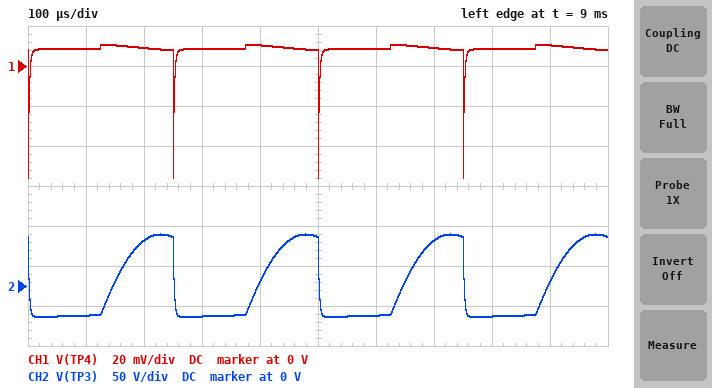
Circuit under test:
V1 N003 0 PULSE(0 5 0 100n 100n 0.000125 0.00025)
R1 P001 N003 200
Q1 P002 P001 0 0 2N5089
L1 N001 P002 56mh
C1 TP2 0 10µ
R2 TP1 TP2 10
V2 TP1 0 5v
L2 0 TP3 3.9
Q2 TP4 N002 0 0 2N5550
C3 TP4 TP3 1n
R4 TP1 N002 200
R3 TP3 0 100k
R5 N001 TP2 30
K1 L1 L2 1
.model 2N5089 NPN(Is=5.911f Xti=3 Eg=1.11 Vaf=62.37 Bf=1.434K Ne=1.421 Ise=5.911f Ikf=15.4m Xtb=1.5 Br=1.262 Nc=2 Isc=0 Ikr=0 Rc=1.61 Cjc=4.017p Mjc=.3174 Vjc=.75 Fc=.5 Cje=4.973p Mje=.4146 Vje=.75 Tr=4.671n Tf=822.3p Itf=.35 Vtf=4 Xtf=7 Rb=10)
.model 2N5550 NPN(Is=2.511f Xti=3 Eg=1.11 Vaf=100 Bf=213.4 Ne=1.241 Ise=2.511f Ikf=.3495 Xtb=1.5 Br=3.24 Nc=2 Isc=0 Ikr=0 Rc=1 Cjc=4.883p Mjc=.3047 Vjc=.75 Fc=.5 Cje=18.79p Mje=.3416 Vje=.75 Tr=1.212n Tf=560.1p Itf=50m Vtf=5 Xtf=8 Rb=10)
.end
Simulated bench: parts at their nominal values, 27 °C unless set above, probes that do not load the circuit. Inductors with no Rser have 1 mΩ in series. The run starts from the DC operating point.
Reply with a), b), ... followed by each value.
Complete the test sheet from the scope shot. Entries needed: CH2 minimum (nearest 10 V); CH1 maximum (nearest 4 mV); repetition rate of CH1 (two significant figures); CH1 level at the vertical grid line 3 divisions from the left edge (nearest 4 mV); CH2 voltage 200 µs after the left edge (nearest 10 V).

a) -40 V
b) 12 mV
c) 4.0 kHz
d) 8 mV
e) 60 V
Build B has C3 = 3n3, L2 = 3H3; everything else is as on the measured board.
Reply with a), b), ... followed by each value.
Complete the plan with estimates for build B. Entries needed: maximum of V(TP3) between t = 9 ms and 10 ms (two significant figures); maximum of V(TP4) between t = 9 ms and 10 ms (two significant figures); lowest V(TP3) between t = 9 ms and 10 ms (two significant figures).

a) 69 V
b) 13 mV
c) -31 V
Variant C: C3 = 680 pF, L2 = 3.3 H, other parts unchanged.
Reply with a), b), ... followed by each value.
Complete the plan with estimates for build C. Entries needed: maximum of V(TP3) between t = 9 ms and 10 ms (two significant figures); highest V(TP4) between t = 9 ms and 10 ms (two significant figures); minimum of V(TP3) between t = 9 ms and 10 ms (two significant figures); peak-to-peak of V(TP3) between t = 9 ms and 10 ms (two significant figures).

a) 57 V
b) 10 mV
c) -37 V
d) 94 V
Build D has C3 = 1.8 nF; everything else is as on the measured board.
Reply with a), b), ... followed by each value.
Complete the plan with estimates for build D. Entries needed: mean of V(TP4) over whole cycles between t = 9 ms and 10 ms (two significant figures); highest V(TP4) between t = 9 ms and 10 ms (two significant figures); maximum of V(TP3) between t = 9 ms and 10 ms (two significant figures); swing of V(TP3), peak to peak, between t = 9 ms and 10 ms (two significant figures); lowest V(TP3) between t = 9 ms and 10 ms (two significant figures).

a) 8.2 mV
b) 12 mV
c) 73 V
d) 110 V
e) -36 V
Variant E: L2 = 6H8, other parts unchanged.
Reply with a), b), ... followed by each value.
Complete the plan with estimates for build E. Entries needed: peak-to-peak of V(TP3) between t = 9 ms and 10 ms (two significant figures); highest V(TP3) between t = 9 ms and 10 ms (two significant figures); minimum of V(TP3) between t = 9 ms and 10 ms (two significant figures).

a) 130 V
b) 84 V
c) -47 V
